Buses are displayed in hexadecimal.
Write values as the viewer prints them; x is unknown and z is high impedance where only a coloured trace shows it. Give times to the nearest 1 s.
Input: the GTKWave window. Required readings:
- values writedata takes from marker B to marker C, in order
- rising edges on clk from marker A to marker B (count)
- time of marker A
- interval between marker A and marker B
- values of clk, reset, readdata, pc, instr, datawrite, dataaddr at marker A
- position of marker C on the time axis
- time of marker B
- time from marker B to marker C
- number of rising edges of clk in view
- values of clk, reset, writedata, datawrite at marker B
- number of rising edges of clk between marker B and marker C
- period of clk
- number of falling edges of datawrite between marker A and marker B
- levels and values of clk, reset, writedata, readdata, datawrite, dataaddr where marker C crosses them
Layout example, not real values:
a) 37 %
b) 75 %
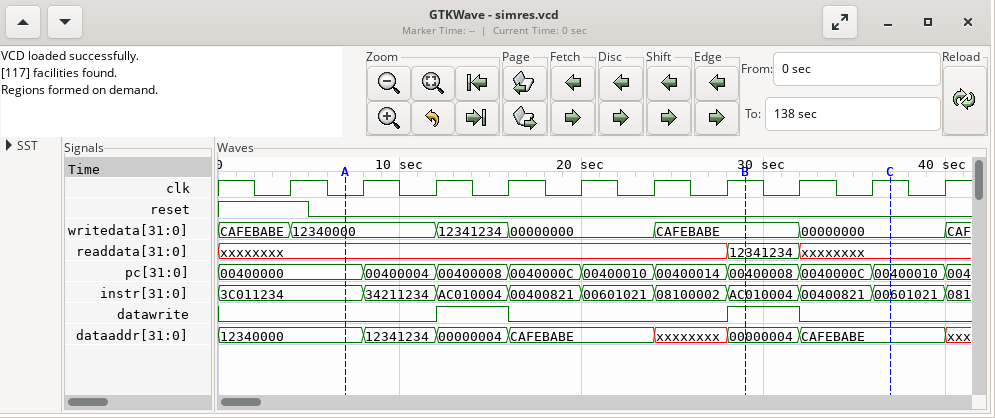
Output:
a) CAFEBABE, 00000000
b) 6
c) 7 s
d) 22 s
e) clk=0, reset=0, readdata=xxxxxxxx, pc=00400000, instr=3C011234, datawrite=0, dataaddr=12340000
f) 37 s
g) 29 s
h) 8 s
i) 10
j) clk=1, reset=0, writedata=CAFEBABE, datawrite=1
k) 2
l) 4 s
m) 1
n) clk=1, reset=0, writedata=00000000, readdata=xxxxxxxx, datawrite=0, dataaddr=CAFEBABE
